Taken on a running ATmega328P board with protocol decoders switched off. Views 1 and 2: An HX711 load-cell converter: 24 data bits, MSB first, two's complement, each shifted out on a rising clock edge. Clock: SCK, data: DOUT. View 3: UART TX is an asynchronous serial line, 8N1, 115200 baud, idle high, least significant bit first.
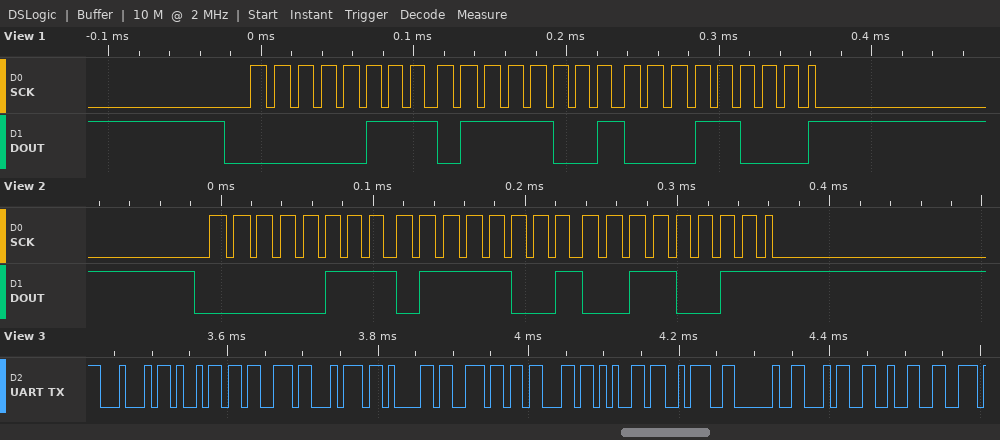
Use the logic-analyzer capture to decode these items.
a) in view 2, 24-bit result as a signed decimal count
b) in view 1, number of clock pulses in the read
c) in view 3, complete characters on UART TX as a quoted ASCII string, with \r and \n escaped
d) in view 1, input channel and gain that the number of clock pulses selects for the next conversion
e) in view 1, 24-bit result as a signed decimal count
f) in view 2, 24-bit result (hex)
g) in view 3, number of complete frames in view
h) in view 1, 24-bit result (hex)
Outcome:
489779
25
"Distance: 42"
channel A, gain 128
489752
0x077933
12
0x077918
